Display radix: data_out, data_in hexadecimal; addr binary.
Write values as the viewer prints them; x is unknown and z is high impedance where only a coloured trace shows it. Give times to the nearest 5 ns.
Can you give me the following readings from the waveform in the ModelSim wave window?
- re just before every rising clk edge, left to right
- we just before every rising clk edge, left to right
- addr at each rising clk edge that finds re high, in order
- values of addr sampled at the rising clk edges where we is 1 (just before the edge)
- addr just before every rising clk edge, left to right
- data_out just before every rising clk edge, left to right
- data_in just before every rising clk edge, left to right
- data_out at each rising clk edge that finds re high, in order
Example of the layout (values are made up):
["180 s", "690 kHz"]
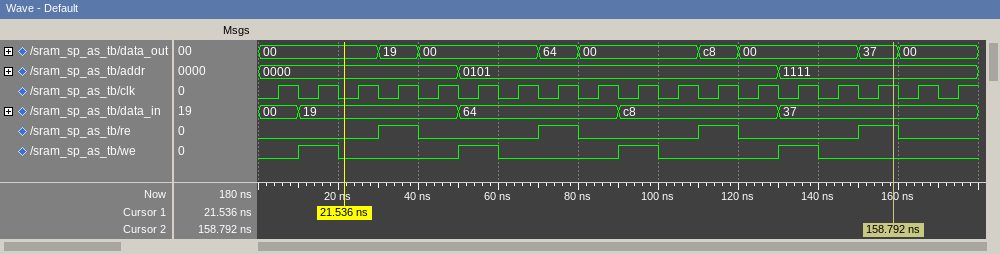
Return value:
["0 0 0 1 0 0 0 1 0 0 0 1 0 0 0 1 0 0", "0 1 0 0 0 1 0 0 0 1 0 0 0 1 0 0 0 0", "0000, 0101, 0101, 1111", "0000, 0101, 0101, 1111", "0000, 0000, 0000, 0000, 0000, 0101, 0101, 0101, 0101, 0101, 0101, 0101, 0101, 1111, 1111, 1111, 1111, 1111", "00, 00, 00, 19, 00, 00, 00, 64, 00, 00, 00, c8, 00, 00, 00, 37, 00, 00", "00, 19, 19, 19, 19, 64, 64, 64, 64, c8, c8, c8, c8, 37, 37, 37, 37, 37", "19, 64, c8, 37"]
